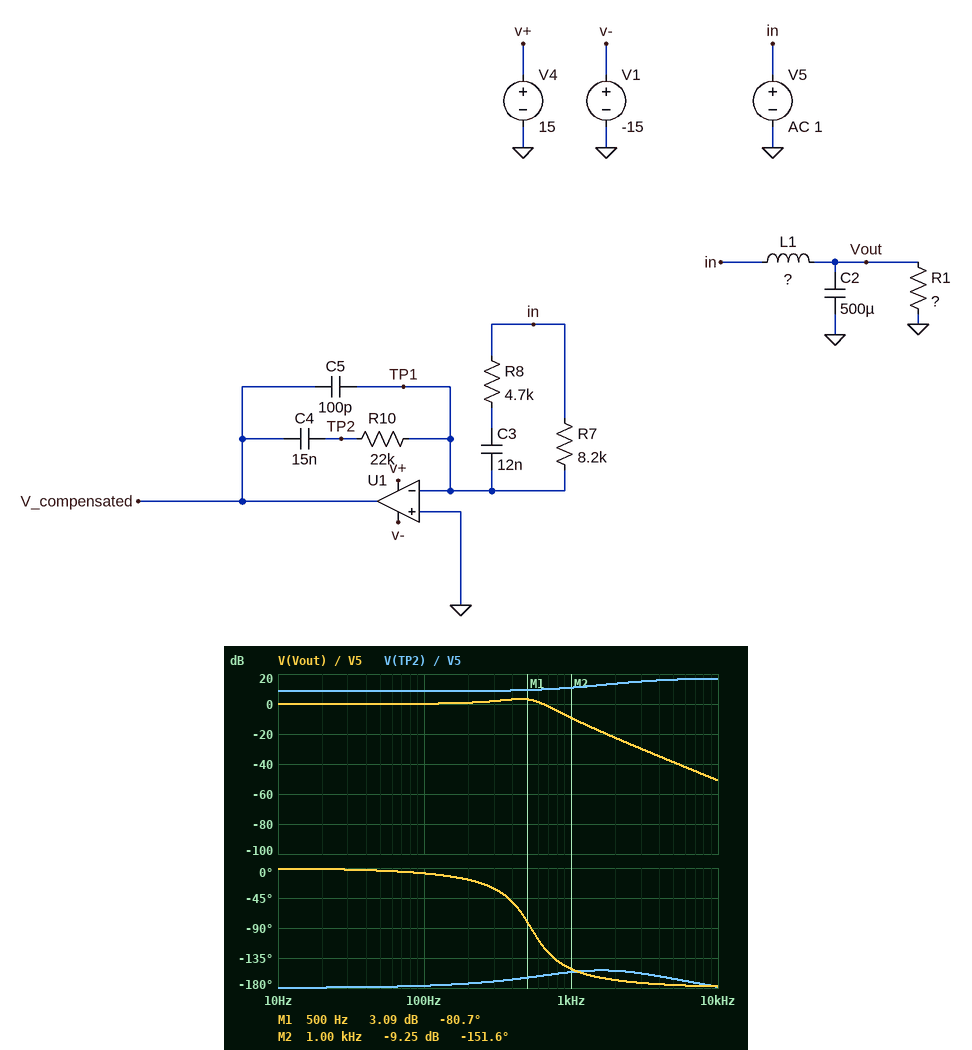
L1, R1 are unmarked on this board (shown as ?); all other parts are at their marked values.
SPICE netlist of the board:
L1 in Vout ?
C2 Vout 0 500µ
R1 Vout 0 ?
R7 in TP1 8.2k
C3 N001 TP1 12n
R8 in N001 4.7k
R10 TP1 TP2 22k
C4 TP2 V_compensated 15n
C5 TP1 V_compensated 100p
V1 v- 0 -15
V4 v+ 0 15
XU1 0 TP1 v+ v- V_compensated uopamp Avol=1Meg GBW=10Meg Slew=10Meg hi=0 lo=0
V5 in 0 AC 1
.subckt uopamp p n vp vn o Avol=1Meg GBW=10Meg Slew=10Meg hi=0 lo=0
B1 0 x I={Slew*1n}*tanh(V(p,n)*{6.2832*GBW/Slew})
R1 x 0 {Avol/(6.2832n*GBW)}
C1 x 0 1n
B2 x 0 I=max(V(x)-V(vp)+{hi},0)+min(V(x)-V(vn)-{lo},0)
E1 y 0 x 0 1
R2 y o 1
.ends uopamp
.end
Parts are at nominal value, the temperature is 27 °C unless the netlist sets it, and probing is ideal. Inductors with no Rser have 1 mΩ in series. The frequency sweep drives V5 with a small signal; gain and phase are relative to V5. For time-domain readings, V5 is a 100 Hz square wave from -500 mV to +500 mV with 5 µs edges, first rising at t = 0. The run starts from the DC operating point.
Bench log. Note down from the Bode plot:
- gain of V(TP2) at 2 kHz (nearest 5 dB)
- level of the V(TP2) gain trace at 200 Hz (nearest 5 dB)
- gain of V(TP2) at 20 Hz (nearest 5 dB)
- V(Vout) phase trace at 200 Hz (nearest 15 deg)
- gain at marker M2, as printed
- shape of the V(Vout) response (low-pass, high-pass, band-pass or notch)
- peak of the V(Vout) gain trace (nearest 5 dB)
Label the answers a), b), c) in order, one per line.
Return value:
a) 15 dB
b) 10 dB
c) 10 dB
d) -15 deg
e) -9.25 dB
f) low-pass
g) 5 dB
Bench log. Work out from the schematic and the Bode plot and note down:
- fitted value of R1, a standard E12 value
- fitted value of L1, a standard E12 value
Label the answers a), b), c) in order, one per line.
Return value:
a) 0.82 Ω
b) 180 µH
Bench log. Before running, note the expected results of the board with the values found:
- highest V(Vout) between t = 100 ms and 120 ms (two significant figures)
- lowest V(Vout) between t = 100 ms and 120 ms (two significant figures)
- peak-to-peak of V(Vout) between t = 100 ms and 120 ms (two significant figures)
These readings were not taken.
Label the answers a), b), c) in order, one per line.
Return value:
a) 790 mV
b) -790 mV
c) 1.6 V
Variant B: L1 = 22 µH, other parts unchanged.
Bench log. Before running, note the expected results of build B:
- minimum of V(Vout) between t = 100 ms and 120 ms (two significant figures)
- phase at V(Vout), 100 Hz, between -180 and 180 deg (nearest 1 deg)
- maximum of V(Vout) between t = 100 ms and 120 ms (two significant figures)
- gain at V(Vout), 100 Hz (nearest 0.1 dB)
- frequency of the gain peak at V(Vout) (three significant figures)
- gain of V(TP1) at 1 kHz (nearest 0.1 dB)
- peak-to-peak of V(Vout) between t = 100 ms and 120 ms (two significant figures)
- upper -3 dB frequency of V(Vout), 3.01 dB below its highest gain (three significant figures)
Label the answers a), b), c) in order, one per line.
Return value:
a) -1.2 V
b) -1 deg
c) 1.2 V
d) 0 dB
e) 1.49 kHz
f) -68.2 dB
g) 2.3 V
h) 1.68 kHz
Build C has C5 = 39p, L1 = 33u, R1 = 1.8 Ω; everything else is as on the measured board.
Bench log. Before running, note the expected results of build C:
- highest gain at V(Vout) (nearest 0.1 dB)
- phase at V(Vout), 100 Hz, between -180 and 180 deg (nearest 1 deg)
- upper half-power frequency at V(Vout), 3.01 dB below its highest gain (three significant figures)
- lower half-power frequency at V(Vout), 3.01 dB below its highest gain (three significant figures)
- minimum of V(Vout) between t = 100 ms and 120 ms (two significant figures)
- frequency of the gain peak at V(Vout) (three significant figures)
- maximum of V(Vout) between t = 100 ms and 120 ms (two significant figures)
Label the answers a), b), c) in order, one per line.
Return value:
a) 16.7 dB
b) -1 deg
c) 1.32 kHz
d) 1.14 kHz
e) -1.3 V
f) 1.23 kHz
g) 1.3 V
